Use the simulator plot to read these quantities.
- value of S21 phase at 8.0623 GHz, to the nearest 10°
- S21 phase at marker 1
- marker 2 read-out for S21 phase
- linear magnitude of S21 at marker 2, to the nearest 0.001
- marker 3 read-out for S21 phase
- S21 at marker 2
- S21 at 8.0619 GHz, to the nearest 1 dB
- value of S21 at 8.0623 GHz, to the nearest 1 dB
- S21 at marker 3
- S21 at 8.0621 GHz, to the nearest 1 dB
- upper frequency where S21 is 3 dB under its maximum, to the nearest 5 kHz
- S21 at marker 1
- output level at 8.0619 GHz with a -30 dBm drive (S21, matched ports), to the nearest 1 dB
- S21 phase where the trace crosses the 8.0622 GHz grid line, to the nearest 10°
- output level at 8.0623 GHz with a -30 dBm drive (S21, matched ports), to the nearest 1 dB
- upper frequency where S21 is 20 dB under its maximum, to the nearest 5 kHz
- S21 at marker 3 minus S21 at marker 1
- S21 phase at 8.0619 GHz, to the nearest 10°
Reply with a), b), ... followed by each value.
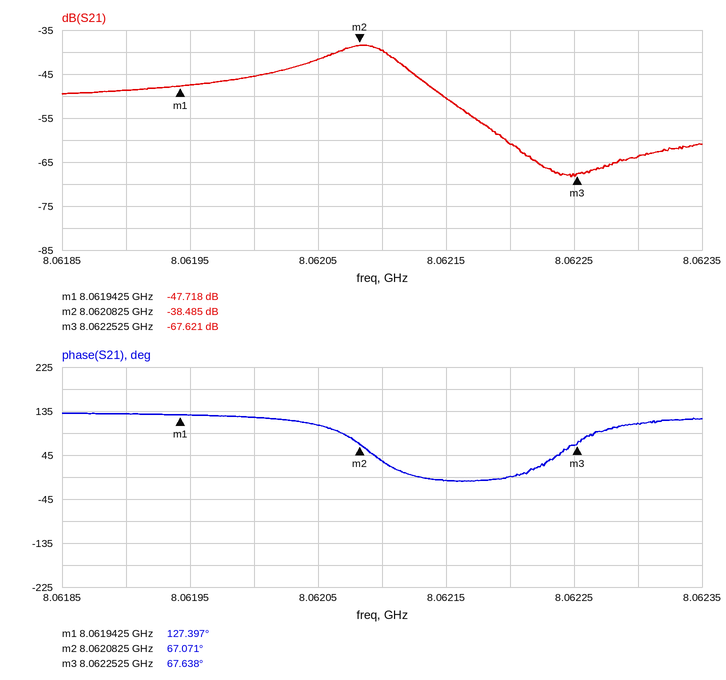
a) 110°
b) 127.397°
c) 67.071°
d) 0.012
e) 67.638°
f) -38.485 dB
g) -49 dB
h) -64 dB
i) -67.621 dB
j) -40 dB
k) 8.062110 GHz
l) -47.718 dB
m) -79 dBm
n) 0°
o) -94 dBm
p) 8.062190 GHz
q) -19.903 dB
r) 130°
